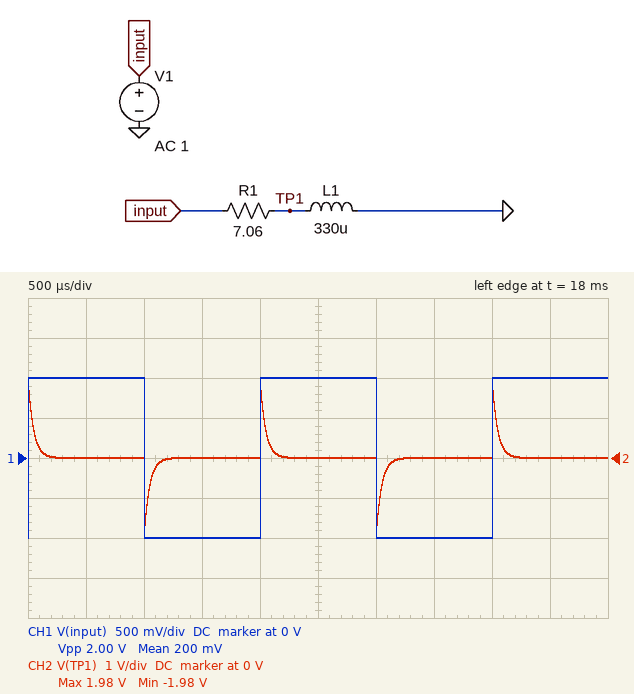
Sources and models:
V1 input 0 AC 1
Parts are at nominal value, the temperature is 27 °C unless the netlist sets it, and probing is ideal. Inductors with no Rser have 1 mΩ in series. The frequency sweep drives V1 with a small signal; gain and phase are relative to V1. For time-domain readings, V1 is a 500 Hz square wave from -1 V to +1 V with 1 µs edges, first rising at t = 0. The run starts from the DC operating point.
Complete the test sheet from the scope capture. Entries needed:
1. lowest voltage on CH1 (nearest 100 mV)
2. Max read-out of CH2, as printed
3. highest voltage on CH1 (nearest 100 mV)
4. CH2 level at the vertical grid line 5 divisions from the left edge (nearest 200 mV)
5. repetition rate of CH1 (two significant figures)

-1.0 V
1.98 V
1.0 V
0 V
500 Hz
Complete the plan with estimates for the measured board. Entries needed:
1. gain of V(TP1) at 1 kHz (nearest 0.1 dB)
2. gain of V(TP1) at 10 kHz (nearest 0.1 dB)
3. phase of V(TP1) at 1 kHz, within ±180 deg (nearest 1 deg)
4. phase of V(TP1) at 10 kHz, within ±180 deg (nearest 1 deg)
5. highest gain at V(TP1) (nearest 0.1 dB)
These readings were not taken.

-11.0 dB
-0.5 dB
74 deg
19 deg
0 dB
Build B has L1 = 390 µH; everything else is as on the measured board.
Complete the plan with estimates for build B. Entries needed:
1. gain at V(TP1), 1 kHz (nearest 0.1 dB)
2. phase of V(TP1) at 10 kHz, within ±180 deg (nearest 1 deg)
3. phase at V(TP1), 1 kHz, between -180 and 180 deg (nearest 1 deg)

-9.7 dB
16 deg
71 deg
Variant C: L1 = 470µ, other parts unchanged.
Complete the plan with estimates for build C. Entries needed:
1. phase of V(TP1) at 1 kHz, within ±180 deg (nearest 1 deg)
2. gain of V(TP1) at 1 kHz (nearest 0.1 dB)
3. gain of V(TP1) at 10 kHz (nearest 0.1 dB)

67 deg
-8.3 dB
-0.2 dB
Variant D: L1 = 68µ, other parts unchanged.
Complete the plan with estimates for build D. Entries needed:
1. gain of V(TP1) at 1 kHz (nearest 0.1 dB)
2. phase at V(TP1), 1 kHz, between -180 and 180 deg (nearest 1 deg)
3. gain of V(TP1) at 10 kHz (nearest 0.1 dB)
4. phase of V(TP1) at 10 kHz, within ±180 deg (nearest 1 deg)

-24.4 dB
86 deg
-5.7 dB
59 deg
